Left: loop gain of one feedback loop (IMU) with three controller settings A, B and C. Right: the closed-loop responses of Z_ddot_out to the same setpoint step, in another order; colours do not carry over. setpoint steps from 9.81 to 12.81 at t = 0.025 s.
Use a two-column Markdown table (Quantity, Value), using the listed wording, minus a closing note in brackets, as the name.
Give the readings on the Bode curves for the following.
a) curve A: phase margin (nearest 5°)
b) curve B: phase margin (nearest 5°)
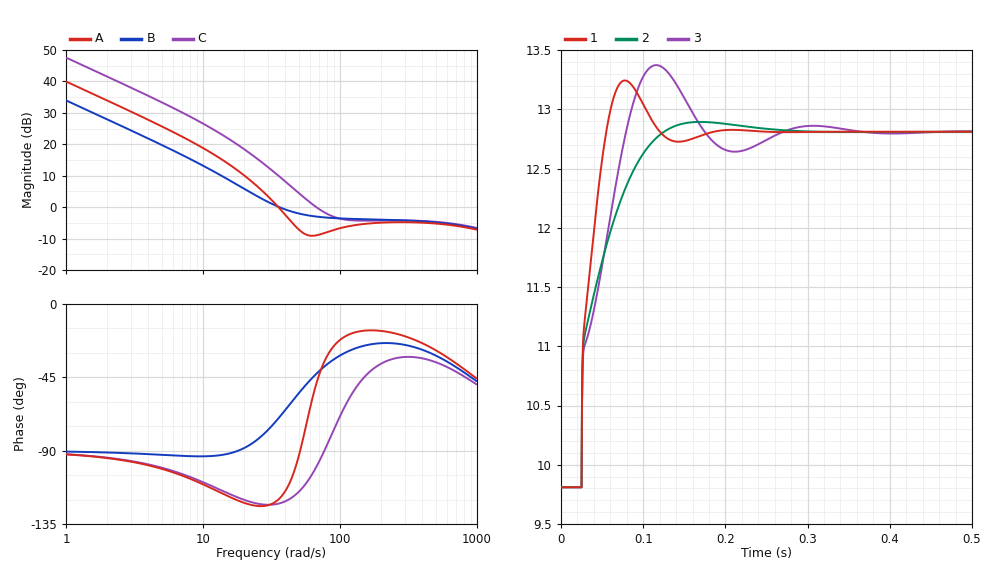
| Quantity | Value |
|---|---|
| curve A: phase margin | 60° |
| curve B: phase margin | 110° |
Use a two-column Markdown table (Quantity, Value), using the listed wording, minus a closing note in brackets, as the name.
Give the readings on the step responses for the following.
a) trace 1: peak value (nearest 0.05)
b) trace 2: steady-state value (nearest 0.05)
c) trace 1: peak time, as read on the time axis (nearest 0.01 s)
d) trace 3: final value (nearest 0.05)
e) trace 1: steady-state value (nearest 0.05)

| Quantity | Value |
|---|---|
| trace 1: peak value | 13.25 |
| trace 2: steady-state value | 12.80 |
| trace 1: peak time, as read on the time axis | 0.08 s |
| trace 3: final value | 12.80 |
| trace 1: steady-state value | 12.80 |
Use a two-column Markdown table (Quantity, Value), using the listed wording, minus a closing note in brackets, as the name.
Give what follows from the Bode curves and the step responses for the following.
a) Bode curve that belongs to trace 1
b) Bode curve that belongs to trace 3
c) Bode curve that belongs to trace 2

| Quantity | Value |
|---|---|
| Bode curve that belongs to trace 1 | C |
| Bode curve that belongs to trace 3 | A |
| Bode curve that belongs to trace 2 | B |
